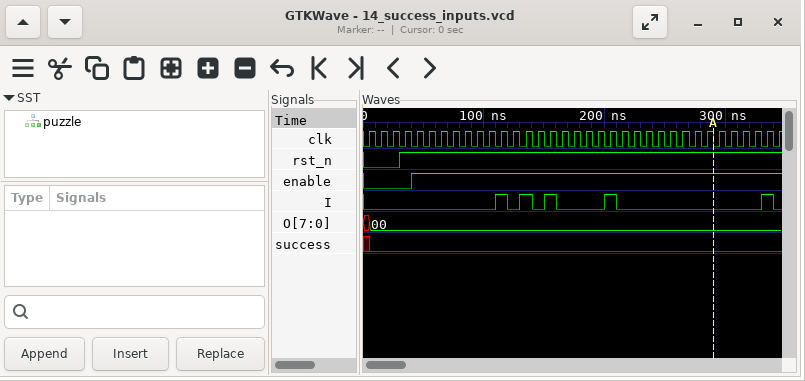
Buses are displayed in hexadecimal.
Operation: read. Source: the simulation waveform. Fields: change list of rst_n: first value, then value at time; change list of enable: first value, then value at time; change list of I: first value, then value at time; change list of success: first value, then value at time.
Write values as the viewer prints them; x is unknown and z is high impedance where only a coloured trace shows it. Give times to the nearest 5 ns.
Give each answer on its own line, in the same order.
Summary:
0, 1 at 30 ns
0, 1 at 40 ns
0, 1 at 110 ns, 0 at 120 ns, 1 at 130 ns, 0 at 140 ns, 1 at 150 ns, 0 at 160 ns, 1 at 200 ns, 0 at 210 ns, 1 at 330 ns, 0 at 340 ns
x, 0 at 5 ns
